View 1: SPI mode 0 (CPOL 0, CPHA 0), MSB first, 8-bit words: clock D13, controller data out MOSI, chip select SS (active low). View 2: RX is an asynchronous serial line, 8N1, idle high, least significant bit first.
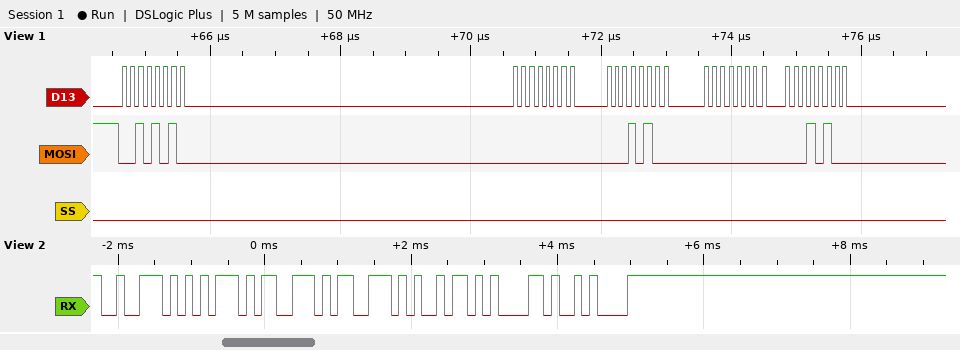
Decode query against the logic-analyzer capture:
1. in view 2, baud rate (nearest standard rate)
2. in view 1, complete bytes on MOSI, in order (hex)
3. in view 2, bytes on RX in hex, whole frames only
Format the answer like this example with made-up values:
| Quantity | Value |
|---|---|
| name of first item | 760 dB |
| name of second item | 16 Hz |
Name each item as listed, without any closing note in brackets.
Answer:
| Quantity | Value |
|---|---|
| in view 2, baud rate | 9600 baud |
| in view 1, complete bytes on MOSI, in order | 0x2A 0x00 0x14 0x00 0x14 |
| in view 2, bytes on RX in hex, whole frames only | 72 75 73 73 69 61 0A |
